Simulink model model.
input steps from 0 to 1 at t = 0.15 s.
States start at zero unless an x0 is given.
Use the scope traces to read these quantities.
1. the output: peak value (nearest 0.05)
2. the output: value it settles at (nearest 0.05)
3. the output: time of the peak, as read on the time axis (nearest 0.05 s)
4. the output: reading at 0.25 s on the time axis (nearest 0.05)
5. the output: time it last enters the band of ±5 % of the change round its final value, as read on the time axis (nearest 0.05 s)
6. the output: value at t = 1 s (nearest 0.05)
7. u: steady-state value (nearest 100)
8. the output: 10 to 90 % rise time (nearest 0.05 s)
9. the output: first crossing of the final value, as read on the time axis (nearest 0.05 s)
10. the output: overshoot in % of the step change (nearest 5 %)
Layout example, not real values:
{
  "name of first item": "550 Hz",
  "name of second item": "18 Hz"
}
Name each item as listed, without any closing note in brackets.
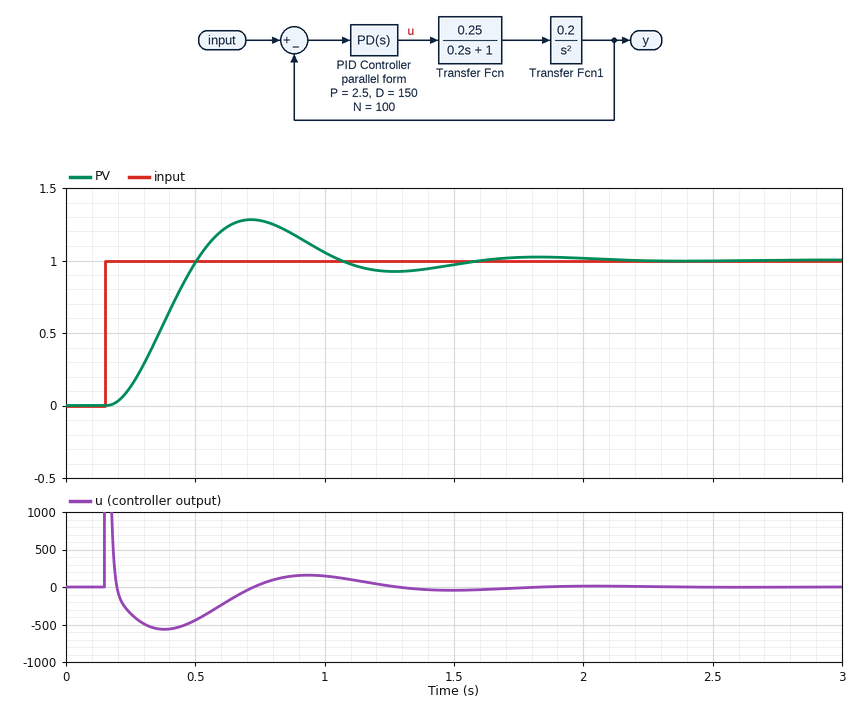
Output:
{
  "the output: peak value": "1.30",
  "the output: value it settles at": "1.00",
  "the output: time of the peak, as read on the time axis": "0.70 s",
  "the output: reading at 0.25 s on the time axis": "0.15",
  "the output: time it last enters the band of ±5 % of the change round its final value, as read on the time axis": "1.45 s",
  "the output: value at t = 1 s": "1.05",
  "u: steady-state value": "0",
  "the output: 10 to 90 % rise time": "0.25 s",
  "the output: first crossing of the final value, as read on the time axis": "0.50 s",
  "the output: overshoot in % of the step change": "30 %"
}
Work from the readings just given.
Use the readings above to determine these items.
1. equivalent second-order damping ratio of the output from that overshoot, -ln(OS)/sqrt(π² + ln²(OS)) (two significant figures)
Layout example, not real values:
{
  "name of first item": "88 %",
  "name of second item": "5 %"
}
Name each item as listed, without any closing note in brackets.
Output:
{
  "equivalent second-order damping ratio of the output from that overshoot, -ln(OS)/sqrt(π² + ln²(OS))": "0.36"
}
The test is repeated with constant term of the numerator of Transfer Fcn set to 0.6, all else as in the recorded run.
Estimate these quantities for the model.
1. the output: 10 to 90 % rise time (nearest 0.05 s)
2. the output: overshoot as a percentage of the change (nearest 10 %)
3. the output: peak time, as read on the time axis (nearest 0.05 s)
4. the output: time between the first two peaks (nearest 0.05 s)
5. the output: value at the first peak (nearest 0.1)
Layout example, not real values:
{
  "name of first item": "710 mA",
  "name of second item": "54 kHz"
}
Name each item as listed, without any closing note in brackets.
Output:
{
  "the output: 10 to 90 % rise time": "0.15 s",
  "the output: overshoot as a percentage of the change": "50 %",
  "the output: peak time, as read on the time axis": "0.50 s",
  "the output: time between the first two peaks": "0.70 s",
  "the output: value at the first peak": "1.5"
}
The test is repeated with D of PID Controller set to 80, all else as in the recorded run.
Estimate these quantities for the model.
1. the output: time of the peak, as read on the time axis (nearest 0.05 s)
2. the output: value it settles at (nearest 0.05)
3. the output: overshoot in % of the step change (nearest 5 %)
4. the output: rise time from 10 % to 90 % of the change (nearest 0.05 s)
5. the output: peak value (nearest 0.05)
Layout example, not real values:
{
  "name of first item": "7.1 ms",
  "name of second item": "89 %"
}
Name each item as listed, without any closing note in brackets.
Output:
{
  "the output: time of the peak, as read on the time axis": "1.00 s",
  "the output: value it settles at": "1.00",
  "the output: overshoot in % of the step change": "15 %",
  "the output: rise time from 10 % to 90 % of the change": "0.40 s",
  "the output: peak value": "1.15"
}
